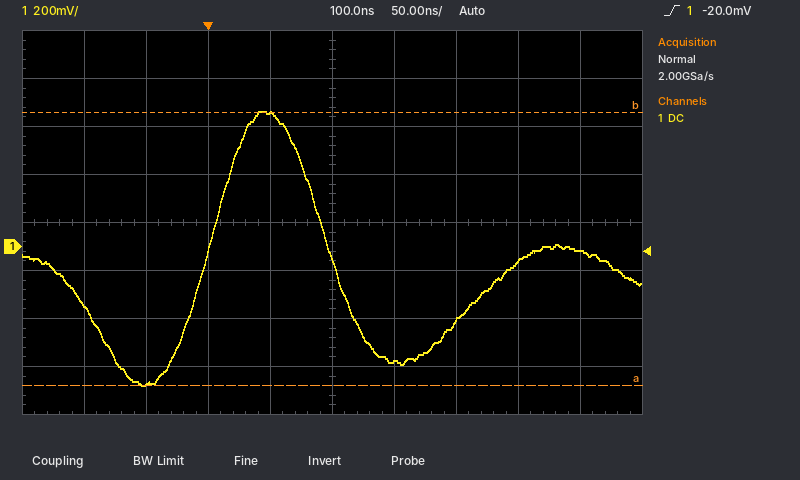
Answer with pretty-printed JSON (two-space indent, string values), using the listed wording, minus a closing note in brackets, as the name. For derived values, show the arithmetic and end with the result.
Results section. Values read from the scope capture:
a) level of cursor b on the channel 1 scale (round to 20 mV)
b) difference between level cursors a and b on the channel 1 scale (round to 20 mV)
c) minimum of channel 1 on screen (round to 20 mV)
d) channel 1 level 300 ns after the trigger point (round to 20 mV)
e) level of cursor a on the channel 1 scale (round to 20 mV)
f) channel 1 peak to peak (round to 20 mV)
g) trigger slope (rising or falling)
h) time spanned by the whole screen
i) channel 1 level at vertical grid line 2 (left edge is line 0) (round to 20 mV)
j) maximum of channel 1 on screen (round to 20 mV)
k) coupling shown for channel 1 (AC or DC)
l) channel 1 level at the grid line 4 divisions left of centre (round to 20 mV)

{
  "level of cursor b on the channel 1 scale": "560 mV",
  "difference between level cursors a and b on the channel 1 scale": "1.14 V",
  "minimum of channel 1 on screen": "-580 mV",
  "channel 1 level 300 ns after the trigger point": "-20 mV",
  "level of cursor a on the channel 1 scale": "-580 mV",
  "channel 1 peak to peak": "560 mV − (-580 mV) = 1.14 V",
  "trigger slope": "rising",
  "time spanned by the whole screen": "500 ns",
  "channel 1 level at vertical grid line 2 (left edge is line 0)": "-580 mV",
  "maximum of channel 1 on screen": "560 mV",
  "coupling shown for channel 1": "DC",
  "channel 1 level at the grid line 4 divisions left of centre": "-240 mV"
}
